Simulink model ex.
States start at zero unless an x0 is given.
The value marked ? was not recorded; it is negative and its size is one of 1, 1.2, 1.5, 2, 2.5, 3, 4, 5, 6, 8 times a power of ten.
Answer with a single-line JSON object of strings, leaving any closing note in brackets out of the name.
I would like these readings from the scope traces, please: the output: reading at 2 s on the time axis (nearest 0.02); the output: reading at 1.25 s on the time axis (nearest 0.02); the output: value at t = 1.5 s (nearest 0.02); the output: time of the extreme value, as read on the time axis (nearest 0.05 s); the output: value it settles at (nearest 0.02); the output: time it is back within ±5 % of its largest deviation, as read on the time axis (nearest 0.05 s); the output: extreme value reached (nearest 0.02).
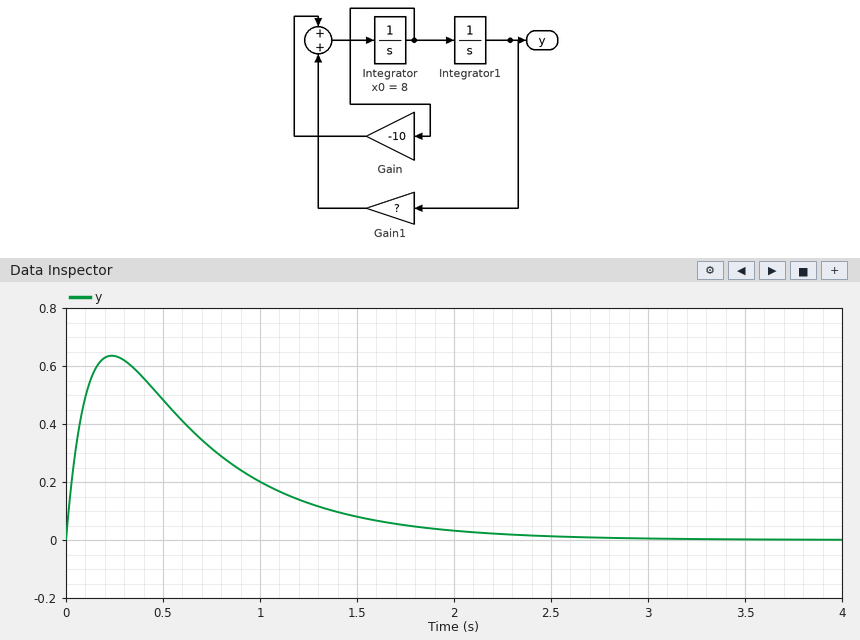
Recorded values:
{"the output: reading at 2 s on the time axis": "0.04", "the output: reading at 1.25 s on the time axis": "0.12", "the output: value at t = 1.5 s": "0.08", "the output: time of the extreme value, as read on the time axis": "0.25 s", "the output: value it settles at": "0.00", "the output: time it is back within ±5 % of its largest deviation, as read on the time axis": "2.00 s", "the output: extreme value reached": "0.64"}
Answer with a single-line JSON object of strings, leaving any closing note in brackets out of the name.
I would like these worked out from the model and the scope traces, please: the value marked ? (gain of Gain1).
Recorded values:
{"the value marked ?": "-15"}
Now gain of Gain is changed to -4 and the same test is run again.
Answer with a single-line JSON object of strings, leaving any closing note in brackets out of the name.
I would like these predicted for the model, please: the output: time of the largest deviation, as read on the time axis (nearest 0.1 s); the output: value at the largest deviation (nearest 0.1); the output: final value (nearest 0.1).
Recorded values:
{"the output: time of the largest deviation, as read on the time axis": "0.3 s", "the output: value at the largest deviation": "1.1", "the output: final value": "0.0"}
